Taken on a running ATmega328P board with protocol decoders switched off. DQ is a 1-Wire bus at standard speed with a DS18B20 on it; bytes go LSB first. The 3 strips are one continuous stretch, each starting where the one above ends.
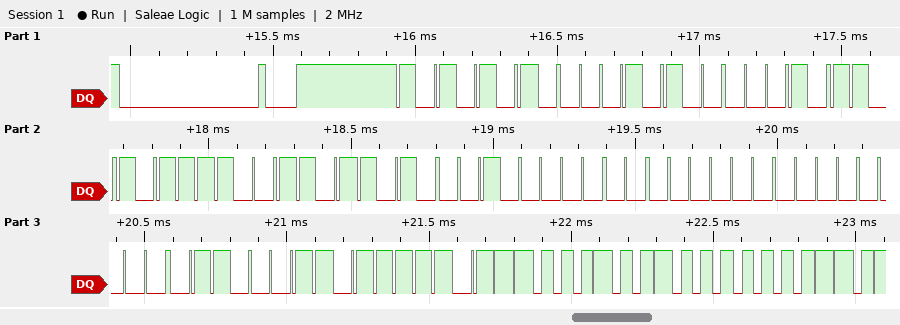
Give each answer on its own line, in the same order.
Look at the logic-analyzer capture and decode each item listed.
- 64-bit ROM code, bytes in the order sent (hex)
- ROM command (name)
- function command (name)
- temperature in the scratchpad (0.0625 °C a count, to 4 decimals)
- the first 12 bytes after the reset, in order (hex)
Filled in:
28 68 3D 5B 04 00 00 C6
Match ROM
Read Scratchpad
18.1875 °C
55 28 68 3D 5B 04 00 00 C6 BE 23 01
